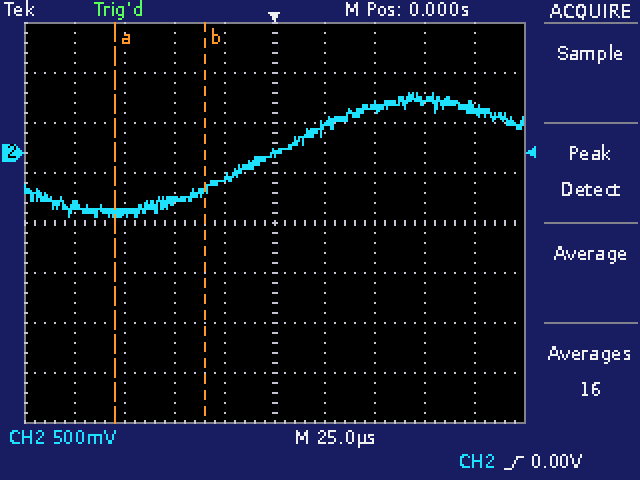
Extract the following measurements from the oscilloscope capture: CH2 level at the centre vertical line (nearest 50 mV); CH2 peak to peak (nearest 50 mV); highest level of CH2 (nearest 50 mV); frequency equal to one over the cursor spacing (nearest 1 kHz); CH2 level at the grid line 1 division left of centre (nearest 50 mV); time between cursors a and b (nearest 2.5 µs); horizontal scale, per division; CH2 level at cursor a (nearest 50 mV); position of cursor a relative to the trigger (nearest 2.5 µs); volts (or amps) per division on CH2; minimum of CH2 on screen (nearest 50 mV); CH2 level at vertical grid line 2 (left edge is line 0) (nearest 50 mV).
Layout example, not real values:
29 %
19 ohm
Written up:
0 mV
1.25 V
600 mV
22 kHz
-250 mV
45.0 µs
25 µs
-600 mV
-80.0 µs
500 mV
-650 mV
-600 mV
